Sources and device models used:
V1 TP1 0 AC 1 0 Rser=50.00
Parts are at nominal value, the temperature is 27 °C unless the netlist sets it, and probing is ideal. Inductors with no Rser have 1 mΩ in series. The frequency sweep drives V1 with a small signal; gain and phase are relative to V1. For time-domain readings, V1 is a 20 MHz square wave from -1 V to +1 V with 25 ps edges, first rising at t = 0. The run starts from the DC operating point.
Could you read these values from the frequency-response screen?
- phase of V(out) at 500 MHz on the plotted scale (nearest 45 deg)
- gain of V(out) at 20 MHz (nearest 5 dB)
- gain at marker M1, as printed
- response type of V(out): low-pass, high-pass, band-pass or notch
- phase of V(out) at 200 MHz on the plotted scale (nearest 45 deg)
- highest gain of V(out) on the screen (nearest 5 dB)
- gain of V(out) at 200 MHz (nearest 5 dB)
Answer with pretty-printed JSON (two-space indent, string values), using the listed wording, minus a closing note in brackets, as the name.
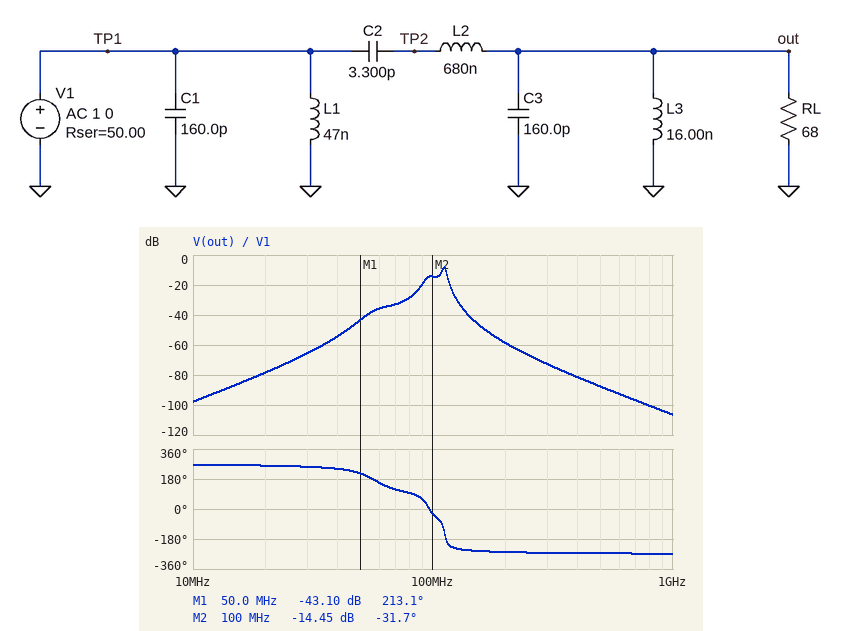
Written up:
{
  "phase of V(out) at 500 MHz on the plotted scale": "-270 deg",
  "gain of V(out) at 20 MHz": "-80 dB",
  "gain at marker M1, as printed": "-43.10 dB",
  "response type of V(out): low-pass, high-pass, band-pass or notch": "band-pass",
  "phase of V(out) at 200 MHz on the plotted scale": "-270 deg",
  "highest gain of V(out) on the screen": "-10 dB",
  "gain of V(out) at 200 MHz": "-60 dB"
}
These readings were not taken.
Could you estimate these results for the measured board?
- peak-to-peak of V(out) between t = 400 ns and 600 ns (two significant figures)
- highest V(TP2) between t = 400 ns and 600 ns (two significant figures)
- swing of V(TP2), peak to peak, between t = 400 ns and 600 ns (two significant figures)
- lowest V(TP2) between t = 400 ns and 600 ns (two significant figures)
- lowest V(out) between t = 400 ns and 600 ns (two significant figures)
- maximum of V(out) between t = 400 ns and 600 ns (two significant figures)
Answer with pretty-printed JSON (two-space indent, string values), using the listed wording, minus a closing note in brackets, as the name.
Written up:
{
  "peak-to-peak of V(out) between t = 400 ns and 600 ns": "110 mV",
  "highest V(TP2) between t = 400 ns and 600 ns": "560 mV",
  "swing of V(TP2), peak to peak, between t = 400 ns and 600 ns": "1.1 V",
  "lowest V(TP2) between t = 400 ns and 600 ns": "-560 mV",
  "lowest V(out) between t = 400 ns and 600 ns": "-57 mV",
  "maximum of V(out) between t = 400 ns and 600 ns": "57 mV"
}
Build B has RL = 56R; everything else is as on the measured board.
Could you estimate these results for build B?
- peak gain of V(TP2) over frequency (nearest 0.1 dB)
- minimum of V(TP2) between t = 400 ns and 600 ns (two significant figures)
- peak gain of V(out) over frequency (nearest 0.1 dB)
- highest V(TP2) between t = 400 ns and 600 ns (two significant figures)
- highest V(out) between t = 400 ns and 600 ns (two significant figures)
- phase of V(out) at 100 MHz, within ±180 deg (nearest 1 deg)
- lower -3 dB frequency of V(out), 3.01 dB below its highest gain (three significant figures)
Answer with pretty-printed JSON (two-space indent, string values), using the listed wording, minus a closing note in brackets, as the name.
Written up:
{
  "peak gain of V(TP2) over frequency": "12.8 dB",
  "minimum of V(TP2) between t = 400 ns and 600 ns": "-590 mV",
  "peak gain of V(out) over frequency": "-9.5 dB",
  "highest V(TP2) between t = 400 ns and 600 ns": "590 mV",
  "highest V(out) between t = 400 ns and 600 ns": "52 mV",
  "phase of V(out) at 100 MHz, within ±180 deg": "-26 deg",
  "lower -3 dB frequency of V(out), 3.01 dB below its highest gain": "108 MHz"
}
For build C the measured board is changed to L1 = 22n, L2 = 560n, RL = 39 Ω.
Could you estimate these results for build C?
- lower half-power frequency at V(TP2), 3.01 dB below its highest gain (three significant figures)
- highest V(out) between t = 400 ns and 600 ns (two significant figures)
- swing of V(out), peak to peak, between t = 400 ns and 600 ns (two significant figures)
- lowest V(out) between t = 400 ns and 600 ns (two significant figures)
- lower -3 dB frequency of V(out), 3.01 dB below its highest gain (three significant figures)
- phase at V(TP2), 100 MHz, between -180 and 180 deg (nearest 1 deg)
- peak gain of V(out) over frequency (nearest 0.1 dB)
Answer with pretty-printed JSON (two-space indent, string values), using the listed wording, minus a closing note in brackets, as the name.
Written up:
{
  "lower half-power frequency at V(TP2), 3.01 dB below its highest gain": "120 MHz",
  "highest V(out) between t = 400 ns and 600 ns": "41 mV",
  "swing of V(out), peak to peak, between t = 400 ns and 600 ns": "81 mV",
  "lowest V(out) between t = 400 ns and 600 ns": "-41 mV",
  "lower -3 dB frequency of V(out), 3.01 dB below its highest gain": "119 MHz",
  "phase at V(TP2), 100 MHz, between -180 and 180 deg": "99 deg",
  "peak gain of V(out) over frequency": "-7.9 dB"
}
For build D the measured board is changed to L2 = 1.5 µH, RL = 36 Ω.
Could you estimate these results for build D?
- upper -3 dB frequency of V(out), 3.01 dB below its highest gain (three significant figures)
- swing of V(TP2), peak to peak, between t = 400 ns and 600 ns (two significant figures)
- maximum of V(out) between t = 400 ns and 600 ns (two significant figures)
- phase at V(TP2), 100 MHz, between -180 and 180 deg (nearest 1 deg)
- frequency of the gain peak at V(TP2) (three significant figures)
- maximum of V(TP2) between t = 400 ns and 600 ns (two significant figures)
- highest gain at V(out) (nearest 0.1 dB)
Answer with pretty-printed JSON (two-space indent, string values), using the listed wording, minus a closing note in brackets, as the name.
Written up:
{
  "upper -3 dB frequency of V(out), 3.01 dB below its highest gain": "73.5 MHz",
  "swing of V(TP2), peak to peak, between t = 400 ns and 600 ns": "2.2 V",
  "maximum of V(out) between t = 400 ns and 600 ns": "21 mV",
  "phase at V(TP2), 100 MHz, between -180 and 180 deg": "-70 deg",
  "frequency of the gain peak at V(TP2)": "72.2 MHz",
  "maximum of V(TP2) between t = 400 ns and 600 ns": "1.1 V",
  "highest gain at V(out)": "-9.0 dB"
}
